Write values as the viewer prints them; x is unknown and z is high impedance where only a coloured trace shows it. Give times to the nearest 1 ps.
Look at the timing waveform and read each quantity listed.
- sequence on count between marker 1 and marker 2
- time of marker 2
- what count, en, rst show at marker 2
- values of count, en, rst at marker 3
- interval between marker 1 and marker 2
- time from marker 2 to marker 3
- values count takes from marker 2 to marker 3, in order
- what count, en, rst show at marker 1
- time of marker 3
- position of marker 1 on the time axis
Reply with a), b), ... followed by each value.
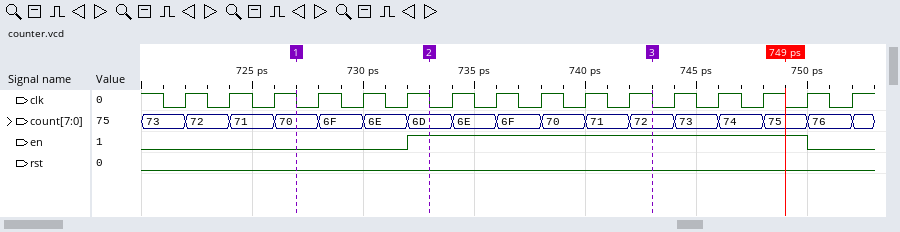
a) 70, 6F, 6E, 6D
b) 733 ps
c) count=6D, en=1, rst=0
d) count=72, en=1, rst=0
e) 6 ps
f) 10 ps
g) 6D, 6E, 6F, 70, 71, 72
h) count=70, en=0, rst=0
i) 743 ps
j) 727 ps
